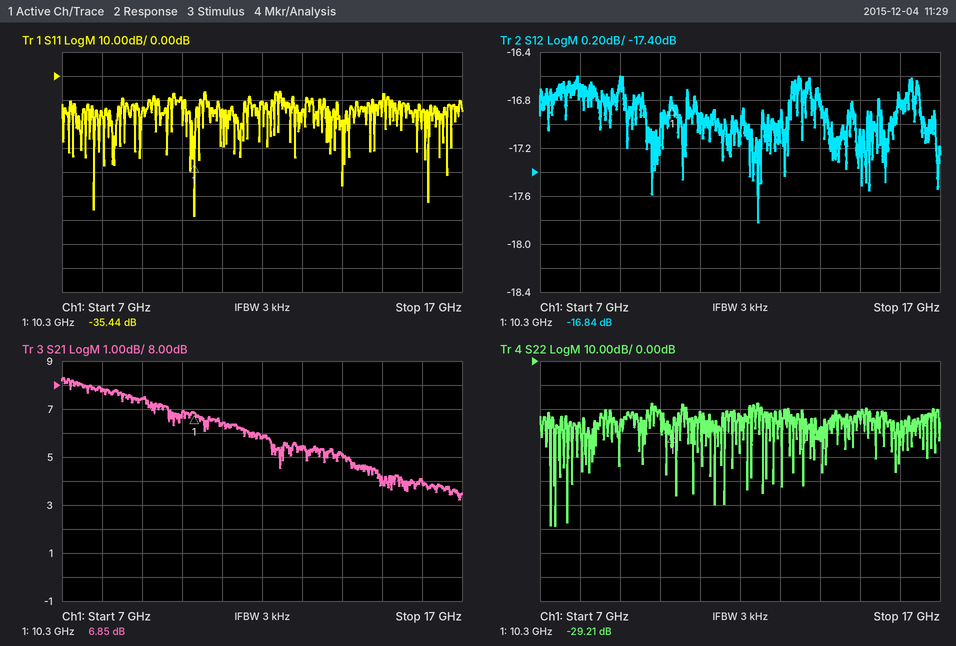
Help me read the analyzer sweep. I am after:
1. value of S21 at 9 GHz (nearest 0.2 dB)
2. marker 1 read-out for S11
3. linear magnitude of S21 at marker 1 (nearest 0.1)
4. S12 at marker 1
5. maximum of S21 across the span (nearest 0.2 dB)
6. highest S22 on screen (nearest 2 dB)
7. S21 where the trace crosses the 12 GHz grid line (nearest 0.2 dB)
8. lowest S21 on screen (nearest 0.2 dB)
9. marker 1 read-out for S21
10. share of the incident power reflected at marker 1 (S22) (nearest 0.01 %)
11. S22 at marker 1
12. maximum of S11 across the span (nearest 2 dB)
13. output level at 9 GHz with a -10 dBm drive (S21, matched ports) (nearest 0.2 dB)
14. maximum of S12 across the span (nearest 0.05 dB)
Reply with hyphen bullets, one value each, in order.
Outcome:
- 7.4 dB
- -35.44 dB
- 2.2
- -16.84 dB
- 8.4 dB
- -18 dB
- 5.8 dB
- 3.2 dB
- 6.85 dB
- 0.12 %
- -29.21 dB
- -6 dB
- -2.6 dBm
- -16.60 dB
